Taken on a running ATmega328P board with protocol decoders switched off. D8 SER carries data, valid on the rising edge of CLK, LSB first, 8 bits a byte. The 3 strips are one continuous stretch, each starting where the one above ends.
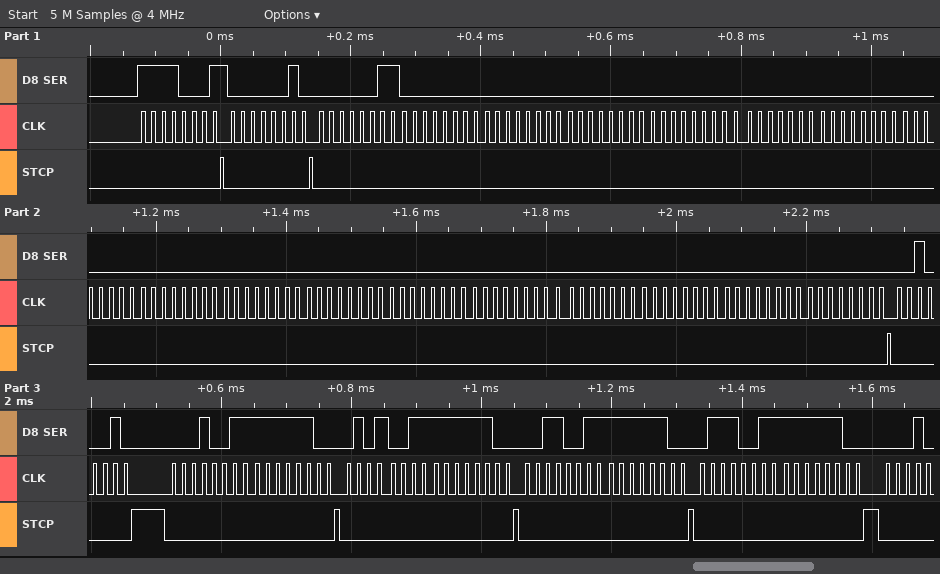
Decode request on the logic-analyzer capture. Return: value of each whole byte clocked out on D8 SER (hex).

8F 40 C0 00 00 00 00 00 00 00 00 00 00 00 00 00 00 00 00 44 C8 3F CA 3F CC 3F CE 3F
